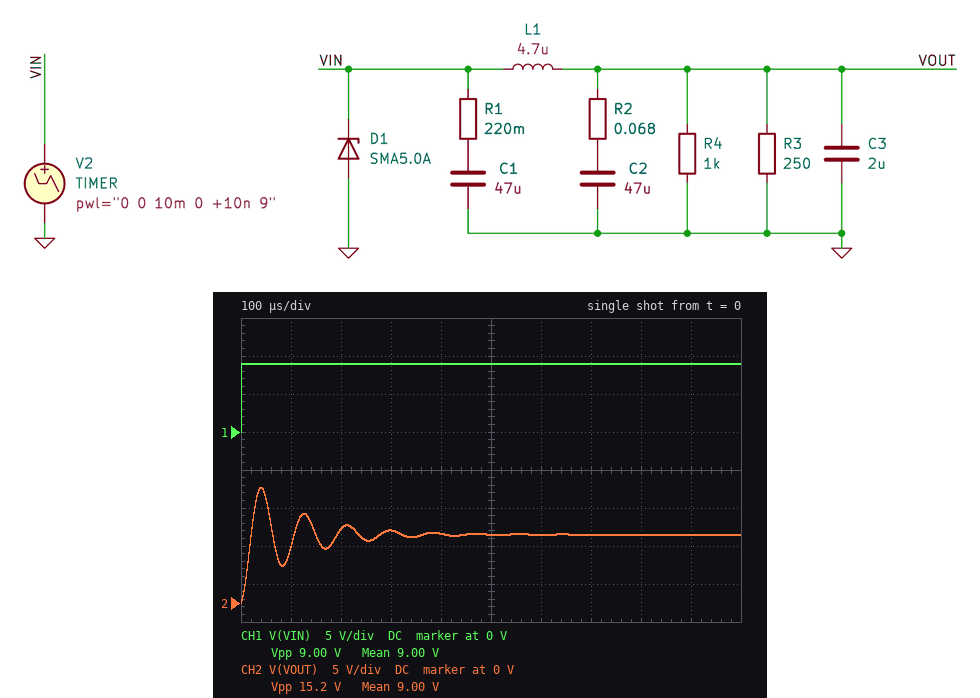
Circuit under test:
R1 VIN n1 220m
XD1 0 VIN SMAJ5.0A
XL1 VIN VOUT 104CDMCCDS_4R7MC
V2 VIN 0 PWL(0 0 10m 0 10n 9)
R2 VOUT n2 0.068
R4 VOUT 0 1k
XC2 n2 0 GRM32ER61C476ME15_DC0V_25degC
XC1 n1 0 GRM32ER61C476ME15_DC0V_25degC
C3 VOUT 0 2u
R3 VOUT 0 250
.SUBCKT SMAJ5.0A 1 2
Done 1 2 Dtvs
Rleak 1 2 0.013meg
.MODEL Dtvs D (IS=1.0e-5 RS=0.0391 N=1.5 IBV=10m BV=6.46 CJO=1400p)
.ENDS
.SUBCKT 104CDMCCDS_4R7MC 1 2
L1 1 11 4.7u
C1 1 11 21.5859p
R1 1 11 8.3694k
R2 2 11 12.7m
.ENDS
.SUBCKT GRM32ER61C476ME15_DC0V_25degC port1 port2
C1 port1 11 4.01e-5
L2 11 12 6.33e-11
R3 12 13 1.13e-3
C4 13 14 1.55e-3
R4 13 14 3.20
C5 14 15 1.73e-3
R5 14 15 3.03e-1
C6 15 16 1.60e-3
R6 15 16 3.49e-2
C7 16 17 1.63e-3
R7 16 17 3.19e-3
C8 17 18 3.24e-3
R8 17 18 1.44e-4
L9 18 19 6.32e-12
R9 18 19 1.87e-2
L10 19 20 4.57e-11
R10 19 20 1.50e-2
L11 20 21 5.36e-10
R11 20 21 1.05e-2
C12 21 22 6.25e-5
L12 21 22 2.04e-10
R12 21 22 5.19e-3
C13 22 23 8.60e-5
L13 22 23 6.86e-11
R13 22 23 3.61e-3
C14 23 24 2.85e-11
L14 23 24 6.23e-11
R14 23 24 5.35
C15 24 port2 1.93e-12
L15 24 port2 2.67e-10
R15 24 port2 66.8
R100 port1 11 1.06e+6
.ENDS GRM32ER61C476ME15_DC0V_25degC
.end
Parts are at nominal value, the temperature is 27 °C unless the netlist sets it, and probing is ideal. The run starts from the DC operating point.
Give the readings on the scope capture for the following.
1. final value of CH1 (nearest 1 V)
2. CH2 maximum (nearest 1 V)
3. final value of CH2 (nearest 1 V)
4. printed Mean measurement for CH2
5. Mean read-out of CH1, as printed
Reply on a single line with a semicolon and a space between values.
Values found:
9 V; 15 V; 9 V; 9.00 V; 9.00 V
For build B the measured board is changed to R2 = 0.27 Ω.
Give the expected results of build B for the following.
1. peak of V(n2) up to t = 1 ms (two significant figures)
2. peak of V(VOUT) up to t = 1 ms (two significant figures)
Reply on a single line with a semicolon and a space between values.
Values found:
11 V; 12 V
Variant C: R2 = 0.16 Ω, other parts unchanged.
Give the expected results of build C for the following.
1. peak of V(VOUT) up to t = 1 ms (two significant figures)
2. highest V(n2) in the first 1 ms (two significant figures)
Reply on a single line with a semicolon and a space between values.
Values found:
14 V; 13 V
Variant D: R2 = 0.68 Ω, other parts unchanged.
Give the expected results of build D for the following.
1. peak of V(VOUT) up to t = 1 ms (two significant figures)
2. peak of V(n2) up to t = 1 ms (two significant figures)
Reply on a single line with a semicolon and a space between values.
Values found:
10 V; 9.0 V
